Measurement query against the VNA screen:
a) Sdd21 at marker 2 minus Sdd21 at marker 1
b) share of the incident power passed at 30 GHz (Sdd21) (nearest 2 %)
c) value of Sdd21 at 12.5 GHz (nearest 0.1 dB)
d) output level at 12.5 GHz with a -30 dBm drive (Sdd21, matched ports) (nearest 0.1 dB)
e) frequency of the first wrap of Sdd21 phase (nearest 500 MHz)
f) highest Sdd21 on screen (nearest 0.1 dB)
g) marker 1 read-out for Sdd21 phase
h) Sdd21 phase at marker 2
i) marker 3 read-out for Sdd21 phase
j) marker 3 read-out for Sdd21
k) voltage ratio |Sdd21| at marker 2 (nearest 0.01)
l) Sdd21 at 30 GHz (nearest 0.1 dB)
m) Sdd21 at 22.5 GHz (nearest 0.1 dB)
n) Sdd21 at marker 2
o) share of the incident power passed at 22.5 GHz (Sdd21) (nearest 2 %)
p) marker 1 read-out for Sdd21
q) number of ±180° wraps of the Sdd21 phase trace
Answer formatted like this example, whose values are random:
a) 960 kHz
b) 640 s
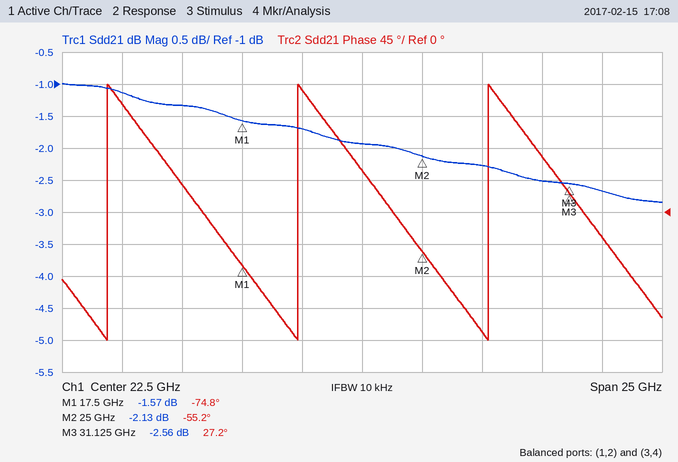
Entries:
a) -0.56 dB
b) 56 %
c) -1.1 dB
d) -31.1 dBm
e) 12.0 GHz
f) -1.0 dB
g) -74.8°
h) -55.2°
i) 27.2°
j) -2.56 dB
k) 0.78
l) -2.5 dB
m) -1.9 dB
n) -2.13 dB
o) 64 %
p) -1.57 dB
q) 3
